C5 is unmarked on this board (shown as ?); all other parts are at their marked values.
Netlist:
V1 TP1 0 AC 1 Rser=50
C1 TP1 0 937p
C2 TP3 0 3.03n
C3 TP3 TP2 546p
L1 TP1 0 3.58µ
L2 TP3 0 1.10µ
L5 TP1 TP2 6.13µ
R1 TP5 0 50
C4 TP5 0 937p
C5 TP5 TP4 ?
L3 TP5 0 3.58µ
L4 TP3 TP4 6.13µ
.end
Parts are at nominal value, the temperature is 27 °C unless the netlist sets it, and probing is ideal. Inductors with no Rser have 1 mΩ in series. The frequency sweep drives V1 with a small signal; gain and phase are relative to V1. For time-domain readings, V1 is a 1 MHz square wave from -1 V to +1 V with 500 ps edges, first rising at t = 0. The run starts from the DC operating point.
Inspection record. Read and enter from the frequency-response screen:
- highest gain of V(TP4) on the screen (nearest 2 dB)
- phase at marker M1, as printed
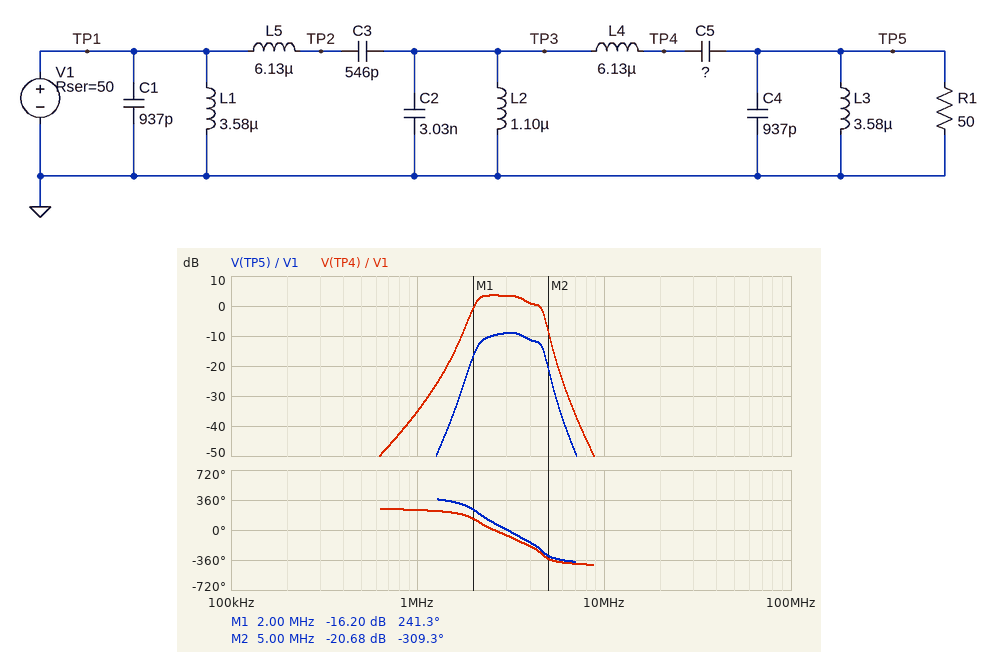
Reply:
4 dB
241.3 deg
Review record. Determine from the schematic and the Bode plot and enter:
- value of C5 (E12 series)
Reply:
270 pF
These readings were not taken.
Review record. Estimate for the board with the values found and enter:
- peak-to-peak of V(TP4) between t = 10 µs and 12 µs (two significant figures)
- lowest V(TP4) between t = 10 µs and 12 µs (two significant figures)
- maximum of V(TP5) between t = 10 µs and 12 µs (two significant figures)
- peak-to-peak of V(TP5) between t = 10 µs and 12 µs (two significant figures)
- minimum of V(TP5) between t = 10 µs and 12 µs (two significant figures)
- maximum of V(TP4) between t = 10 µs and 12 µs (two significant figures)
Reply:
1.4 V
-710 mV
170 mV
340 mV
-170 mV
710 mV
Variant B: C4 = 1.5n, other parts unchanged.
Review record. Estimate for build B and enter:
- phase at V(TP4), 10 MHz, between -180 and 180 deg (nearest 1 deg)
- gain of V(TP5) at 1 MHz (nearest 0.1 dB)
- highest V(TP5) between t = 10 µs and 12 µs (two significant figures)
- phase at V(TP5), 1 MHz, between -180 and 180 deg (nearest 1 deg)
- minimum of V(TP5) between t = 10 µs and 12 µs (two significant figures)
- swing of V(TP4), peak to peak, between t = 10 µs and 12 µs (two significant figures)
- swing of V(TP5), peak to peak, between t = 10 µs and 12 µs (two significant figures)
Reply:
-66 deg
-62.2 dB
140 mV
29 deg
-140 mV
1.5 V
280 mV
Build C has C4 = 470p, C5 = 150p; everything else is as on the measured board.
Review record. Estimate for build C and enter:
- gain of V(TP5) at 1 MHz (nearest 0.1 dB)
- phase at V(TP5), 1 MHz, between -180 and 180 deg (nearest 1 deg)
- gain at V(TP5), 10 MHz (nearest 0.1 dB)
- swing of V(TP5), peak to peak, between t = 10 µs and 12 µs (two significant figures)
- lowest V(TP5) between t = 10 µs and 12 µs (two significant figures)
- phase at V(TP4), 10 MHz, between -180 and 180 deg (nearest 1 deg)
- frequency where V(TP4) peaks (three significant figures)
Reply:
-69.0 dB
34 deg
-62.7 dB
190 mV
-96 mV
-56 deg
2.93 MHz
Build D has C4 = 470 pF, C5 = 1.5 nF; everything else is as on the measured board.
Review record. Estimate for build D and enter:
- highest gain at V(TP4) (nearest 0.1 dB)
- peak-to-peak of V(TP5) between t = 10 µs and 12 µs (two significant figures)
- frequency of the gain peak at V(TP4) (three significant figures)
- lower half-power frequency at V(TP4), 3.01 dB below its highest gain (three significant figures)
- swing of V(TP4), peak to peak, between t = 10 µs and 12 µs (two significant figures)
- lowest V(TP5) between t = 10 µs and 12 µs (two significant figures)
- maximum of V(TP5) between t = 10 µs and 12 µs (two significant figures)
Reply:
-7.6 dB
330 mV
3.36 MHz
2.14 MHz
390 mV
-160 mV
160 mV
